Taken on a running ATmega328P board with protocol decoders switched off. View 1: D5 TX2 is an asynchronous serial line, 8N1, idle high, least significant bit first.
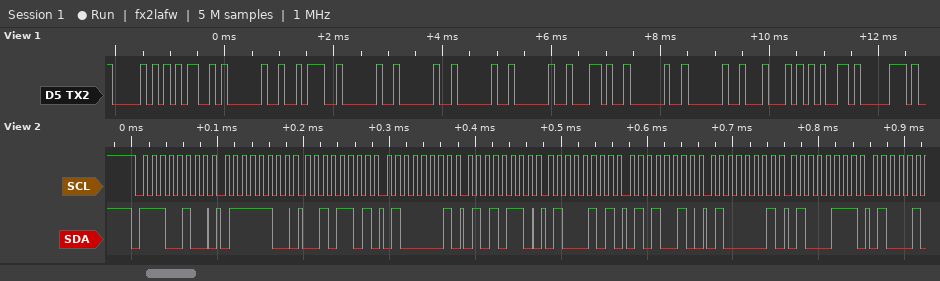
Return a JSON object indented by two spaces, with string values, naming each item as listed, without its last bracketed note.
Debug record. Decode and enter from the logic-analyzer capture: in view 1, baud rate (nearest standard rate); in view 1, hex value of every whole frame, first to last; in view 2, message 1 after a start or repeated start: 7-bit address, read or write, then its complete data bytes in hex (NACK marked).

{
  "in view 1, baud rate": "9600 baud",
  "in view 1, hex value of every whole frame, first to last": "50 4D 20 3A 20 20 20 20 2C 20 20 44 65 70",
  "in view 2, message 1 after a start or repeated start: 7-bit address, read or write, then its complete data bytes in hex": "0x72 write: 7C 2D 41 56 45 52 41 47"
}
